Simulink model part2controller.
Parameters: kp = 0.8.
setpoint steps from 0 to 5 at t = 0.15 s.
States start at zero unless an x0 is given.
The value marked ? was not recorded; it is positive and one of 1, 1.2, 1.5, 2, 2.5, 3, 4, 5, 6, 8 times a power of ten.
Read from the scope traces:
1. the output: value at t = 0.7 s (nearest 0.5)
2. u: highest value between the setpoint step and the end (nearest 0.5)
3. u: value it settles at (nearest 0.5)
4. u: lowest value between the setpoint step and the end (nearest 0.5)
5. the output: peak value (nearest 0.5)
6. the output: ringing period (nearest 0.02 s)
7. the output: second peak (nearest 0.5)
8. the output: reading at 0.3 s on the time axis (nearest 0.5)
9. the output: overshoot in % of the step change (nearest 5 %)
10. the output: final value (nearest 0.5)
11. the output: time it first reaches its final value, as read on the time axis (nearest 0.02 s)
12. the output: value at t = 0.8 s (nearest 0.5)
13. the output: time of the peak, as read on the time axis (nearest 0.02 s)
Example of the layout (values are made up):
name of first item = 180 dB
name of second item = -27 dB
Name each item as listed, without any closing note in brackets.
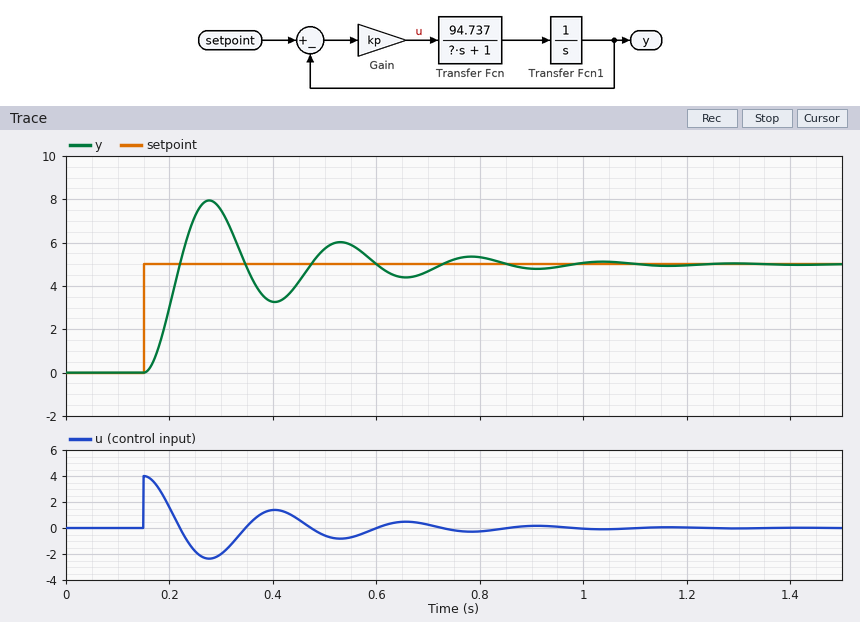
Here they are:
the output: value at t = 0.7 s = 4.5
u: highest value between the setpoint step and the end = 4.0
u: value it settles at = 0.0
u: lowest value between the setpoint step and the end = -2.5
the output: peak value = 8.0
the output: ringing period = 0.26 s
the output: second peak = 6.0
the output: reading at 0.3 s on the time axis = 7.5
the output: overshoot in % of the step change = 60 %
the output: final value = 5.0
the output: time it first reaches its final value, as read on the time axis = 0.22 s
the output: value at t = 0.8 s = 5.5
the output: time of the peak, as read on the time axis = 0.28 s
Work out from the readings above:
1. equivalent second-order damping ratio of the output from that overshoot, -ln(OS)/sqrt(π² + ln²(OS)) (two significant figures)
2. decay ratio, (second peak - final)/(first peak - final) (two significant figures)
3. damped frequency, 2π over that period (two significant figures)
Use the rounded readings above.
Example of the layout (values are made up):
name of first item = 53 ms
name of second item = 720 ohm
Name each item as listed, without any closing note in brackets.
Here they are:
equivalent second-order damping ratio of the output from that overshoot, -ln(OS)/sqrt(π² + ln²(OS)) = 0.16
decay ratio, (second peak - final)/(first peak - final) = 0.33
damped frequency, 2π over that period = 24 rad/s
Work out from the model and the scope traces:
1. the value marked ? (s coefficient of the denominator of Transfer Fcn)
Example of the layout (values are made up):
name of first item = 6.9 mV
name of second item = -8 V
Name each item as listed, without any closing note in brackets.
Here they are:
the value marked ? = 0.12
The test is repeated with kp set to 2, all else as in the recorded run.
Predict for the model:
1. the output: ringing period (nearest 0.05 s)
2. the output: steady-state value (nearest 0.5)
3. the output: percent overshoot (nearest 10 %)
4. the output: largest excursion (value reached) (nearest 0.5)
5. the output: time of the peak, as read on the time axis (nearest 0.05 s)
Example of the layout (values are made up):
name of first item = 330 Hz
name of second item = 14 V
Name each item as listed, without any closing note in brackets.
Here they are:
the output: ringing period = 0.15 s
the output: steady-state value = 5.0
the output: percent overshoot = 70 %
the output: largest excursion (value reached) = 8.5
the output: time of the peak, as read on the time axis = 0.25 s
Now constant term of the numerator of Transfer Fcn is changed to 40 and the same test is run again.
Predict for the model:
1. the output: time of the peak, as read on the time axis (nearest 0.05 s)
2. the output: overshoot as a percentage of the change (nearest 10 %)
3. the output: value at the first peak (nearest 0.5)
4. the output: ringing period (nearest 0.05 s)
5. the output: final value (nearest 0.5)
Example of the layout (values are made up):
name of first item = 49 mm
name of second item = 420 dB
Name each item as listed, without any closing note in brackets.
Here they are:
the output: time of the peak, as read on the time axis = 0.35 s
the output: overshoot as a percentage of the change = 40 %
the output: value at the first peak = 7.0
the output: ringing period = 0.40 s
the output: final value = 5.0
